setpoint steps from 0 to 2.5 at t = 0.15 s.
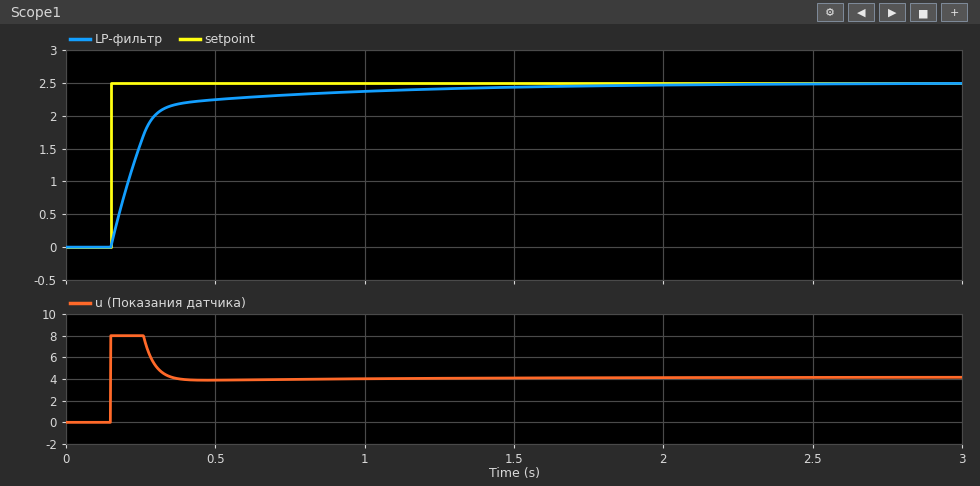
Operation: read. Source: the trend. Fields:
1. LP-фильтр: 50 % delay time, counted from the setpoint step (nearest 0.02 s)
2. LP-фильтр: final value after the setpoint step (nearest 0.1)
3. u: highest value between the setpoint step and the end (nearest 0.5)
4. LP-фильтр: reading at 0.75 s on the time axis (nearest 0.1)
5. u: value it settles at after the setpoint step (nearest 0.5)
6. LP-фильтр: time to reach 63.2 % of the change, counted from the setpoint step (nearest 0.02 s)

0.08 s
2.5
8.0
2.3
4.0
0.10 s
